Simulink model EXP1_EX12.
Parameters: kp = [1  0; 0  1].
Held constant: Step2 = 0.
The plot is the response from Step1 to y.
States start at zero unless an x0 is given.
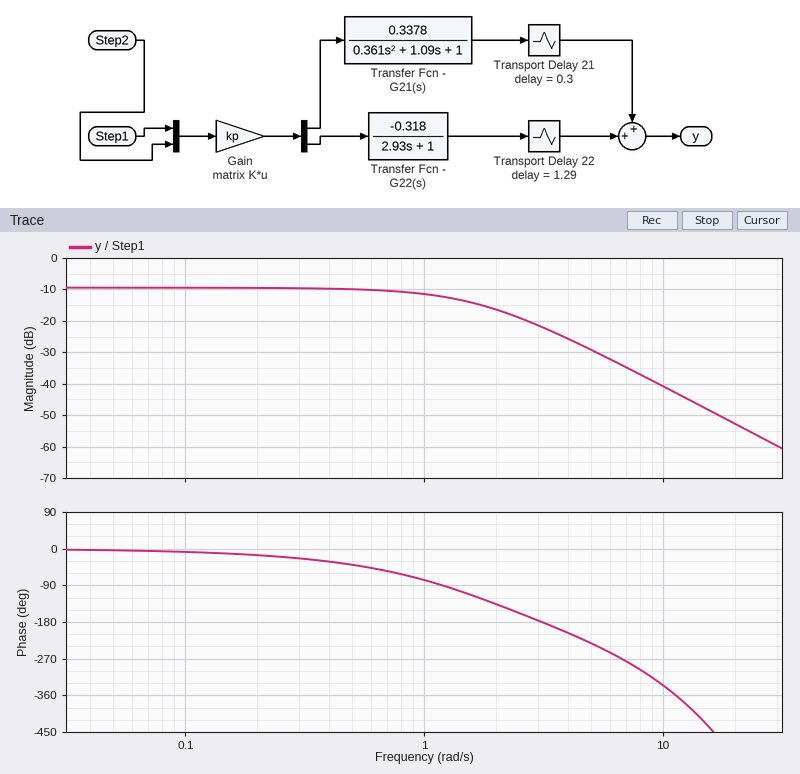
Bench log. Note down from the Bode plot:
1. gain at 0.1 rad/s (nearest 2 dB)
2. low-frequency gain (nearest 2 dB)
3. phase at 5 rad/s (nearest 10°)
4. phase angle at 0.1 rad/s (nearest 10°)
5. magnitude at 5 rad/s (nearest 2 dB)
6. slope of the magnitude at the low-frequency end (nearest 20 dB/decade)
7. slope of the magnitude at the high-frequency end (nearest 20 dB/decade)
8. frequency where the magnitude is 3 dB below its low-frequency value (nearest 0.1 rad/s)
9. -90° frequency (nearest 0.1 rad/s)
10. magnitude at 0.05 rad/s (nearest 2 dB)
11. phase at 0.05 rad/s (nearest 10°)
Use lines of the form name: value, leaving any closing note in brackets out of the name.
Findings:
gain at 0.1 rad/s: -10 dB
low-frequency gain: -10 dB
phase at 5 rad/s: -230°
phase angle at 0.1 rad/s: -10°
magnitude at 5 rad/s: -30 dB
slope of the magnitude at the low-frequency end: 0 dB/decade
slope of the magnitude at the high-frequency end: -40 dB/decade
frequency where the magnitude is 3 dB below its low-frequency value: 1.2 rad/s
-90° frequency: 1.2 rad/s
magnitude at 0.05 rad/s: -10 dB
phase at 0.05 rad/s: 0°
